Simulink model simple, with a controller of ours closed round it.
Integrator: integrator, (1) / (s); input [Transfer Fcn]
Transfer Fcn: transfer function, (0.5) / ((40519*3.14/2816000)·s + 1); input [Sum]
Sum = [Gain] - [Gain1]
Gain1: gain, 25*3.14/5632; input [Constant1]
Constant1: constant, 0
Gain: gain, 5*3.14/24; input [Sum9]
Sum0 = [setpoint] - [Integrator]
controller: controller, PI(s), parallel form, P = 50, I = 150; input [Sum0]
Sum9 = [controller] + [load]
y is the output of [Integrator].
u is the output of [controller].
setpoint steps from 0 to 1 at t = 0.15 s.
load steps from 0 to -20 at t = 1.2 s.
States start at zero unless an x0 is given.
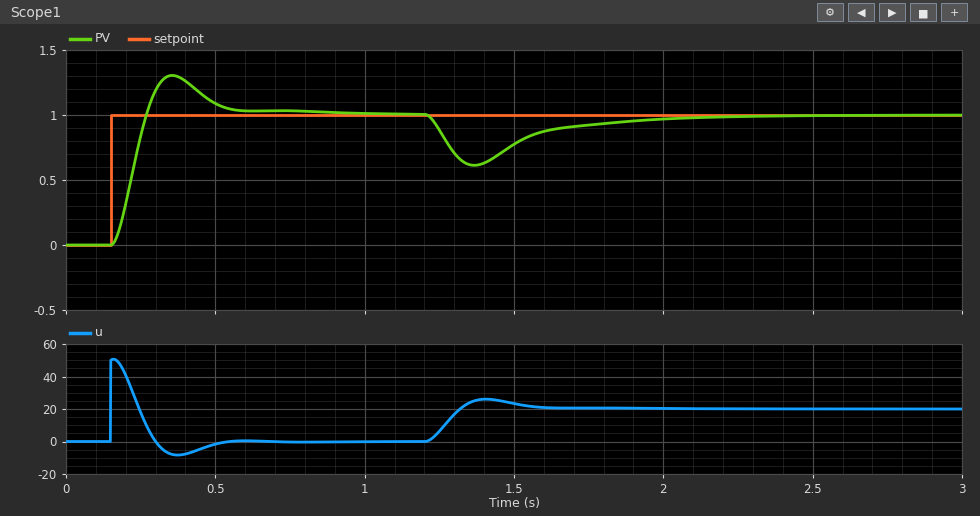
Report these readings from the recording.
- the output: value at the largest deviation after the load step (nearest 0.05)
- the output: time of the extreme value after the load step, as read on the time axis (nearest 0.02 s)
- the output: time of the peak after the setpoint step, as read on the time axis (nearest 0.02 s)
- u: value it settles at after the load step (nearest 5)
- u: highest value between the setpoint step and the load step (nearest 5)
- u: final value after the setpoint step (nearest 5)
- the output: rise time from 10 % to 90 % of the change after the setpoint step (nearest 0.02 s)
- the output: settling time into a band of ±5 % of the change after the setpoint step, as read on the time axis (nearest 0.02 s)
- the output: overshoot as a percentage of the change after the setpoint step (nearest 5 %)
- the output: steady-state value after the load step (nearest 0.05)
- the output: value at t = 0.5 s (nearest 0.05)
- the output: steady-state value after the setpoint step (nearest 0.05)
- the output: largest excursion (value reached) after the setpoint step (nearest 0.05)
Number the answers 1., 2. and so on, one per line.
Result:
1. 0.60
2. 1.36 s
3. 0.36 s
4. 20
5. 50
6. 0
7. 0.08 s
8. 0.54 s
9. 30 %
10. 1.00
11. 1.10
12. 1.00
13. 1.30
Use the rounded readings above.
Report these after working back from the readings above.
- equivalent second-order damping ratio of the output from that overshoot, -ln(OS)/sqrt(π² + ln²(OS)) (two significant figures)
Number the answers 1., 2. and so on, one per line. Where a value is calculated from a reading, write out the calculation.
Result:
1. ln(0.3) = -1.204; 1.204 / sqrt(9.870 + 1.450) = 0.36
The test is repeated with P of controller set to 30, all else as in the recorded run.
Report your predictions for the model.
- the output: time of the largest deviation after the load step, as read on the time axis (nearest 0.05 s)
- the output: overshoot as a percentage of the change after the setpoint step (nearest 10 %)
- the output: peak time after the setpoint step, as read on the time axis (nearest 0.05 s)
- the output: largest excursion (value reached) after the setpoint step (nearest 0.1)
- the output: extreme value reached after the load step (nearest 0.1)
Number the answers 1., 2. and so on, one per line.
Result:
1. 1.40 s
2. 40 %
3. 0.45 s
4. 1.4
5. 0.5
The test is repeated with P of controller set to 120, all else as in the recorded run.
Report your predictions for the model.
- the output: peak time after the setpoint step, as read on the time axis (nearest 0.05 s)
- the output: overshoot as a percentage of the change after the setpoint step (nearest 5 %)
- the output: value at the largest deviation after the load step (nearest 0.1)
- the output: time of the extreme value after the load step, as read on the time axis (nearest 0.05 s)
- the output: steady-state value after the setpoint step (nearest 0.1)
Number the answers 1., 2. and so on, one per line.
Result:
1. 0.25 s
2. 35 %
3. 0.8
4. 1.30 s
5. 1.0
